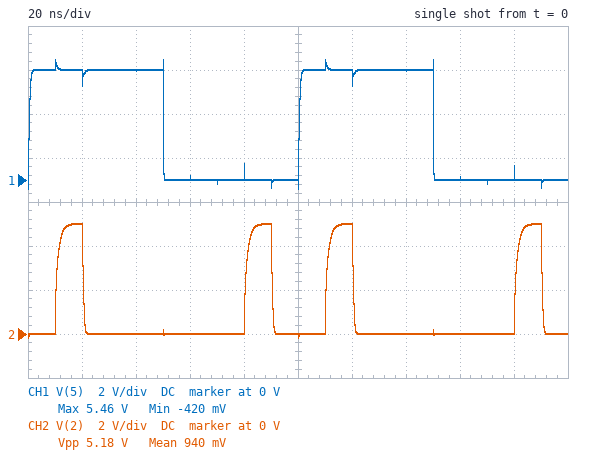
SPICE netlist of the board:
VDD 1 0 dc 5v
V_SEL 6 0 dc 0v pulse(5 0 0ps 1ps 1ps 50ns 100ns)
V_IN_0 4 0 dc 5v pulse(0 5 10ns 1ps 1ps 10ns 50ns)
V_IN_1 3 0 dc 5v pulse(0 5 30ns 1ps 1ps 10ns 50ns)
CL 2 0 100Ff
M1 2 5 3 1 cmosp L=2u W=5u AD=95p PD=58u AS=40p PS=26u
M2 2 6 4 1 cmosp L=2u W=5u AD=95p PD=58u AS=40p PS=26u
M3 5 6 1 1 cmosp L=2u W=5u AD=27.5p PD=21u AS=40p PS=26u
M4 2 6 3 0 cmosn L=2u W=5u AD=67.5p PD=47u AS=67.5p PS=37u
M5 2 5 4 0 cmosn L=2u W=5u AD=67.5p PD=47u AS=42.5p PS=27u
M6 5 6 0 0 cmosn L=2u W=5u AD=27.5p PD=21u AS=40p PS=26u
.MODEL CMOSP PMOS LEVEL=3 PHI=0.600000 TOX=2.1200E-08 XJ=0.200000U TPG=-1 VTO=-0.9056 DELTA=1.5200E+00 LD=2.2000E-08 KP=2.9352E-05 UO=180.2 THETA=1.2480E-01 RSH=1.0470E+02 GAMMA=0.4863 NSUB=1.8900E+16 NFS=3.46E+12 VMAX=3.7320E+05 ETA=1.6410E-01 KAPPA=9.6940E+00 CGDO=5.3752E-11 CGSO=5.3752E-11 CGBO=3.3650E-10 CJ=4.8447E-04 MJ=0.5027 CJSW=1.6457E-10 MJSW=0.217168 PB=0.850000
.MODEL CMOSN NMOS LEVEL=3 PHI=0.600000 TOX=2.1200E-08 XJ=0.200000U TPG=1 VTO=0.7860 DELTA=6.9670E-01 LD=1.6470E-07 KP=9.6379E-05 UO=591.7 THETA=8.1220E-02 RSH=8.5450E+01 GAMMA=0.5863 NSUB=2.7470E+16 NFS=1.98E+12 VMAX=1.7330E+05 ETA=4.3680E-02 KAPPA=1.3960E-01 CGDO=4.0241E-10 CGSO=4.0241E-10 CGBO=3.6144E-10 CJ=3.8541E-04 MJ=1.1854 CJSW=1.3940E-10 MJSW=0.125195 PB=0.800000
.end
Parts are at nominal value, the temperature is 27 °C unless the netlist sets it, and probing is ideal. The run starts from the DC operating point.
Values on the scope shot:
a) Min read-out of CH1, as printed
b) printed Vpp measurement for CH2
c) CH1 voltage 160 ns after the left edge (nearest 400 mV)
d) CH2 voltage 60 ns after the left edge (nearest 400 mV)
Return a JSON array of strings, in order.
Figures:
["-420 mV", "5.18 V", "0 V", "0 V"]
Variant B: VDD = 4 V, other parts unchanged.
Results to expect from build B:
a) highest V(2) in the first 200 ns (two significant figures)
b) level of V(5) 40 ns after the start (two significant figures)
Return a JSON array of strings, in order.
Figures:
["4.5 V", "4.0 V"]
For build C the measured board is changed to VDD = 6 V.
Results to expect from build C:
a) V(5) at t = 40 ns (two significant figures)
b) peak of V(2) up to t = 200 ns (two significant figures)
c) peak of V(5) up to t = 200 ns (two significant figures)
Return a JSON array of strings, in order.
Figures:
["6.0 V", "5.0 V", "6.5 V"]
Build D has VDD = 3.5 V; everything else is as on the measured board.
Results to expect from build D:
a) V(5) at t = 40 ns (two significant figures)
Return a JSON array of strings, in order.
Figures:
["3.5 V"]
